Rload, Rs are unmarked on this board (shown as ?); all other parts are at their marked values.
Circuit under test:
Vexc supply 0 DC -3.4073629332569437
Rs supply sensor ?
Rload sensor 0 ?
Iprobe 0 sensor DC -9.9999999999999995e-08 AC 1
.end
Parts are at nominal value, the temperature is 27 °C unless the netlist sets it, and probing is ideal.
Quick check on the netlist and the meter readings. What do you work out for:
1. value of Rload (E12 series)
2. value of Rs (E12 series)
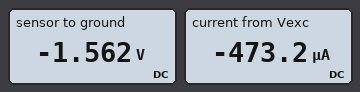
3.3 kΩ
3.9 kΩ
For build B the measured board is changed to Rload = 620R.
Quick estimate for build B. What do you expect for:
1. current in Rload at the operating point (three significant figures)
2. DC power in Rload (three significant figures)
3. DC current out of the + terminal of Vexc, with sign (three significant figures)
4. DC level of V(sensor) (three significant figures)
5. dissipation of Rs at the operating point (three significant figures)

754 µA
352 µW
-754 µA
-467 mV
2.22 mW
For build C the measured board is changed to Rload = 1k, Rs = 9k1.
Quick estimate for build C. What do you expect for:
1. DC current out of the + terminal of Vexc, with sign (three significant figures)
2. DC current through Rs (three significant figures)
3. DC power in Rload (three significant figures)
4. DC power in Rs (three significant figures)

-337 µA
337 µA
114 µW
1.04 mW
